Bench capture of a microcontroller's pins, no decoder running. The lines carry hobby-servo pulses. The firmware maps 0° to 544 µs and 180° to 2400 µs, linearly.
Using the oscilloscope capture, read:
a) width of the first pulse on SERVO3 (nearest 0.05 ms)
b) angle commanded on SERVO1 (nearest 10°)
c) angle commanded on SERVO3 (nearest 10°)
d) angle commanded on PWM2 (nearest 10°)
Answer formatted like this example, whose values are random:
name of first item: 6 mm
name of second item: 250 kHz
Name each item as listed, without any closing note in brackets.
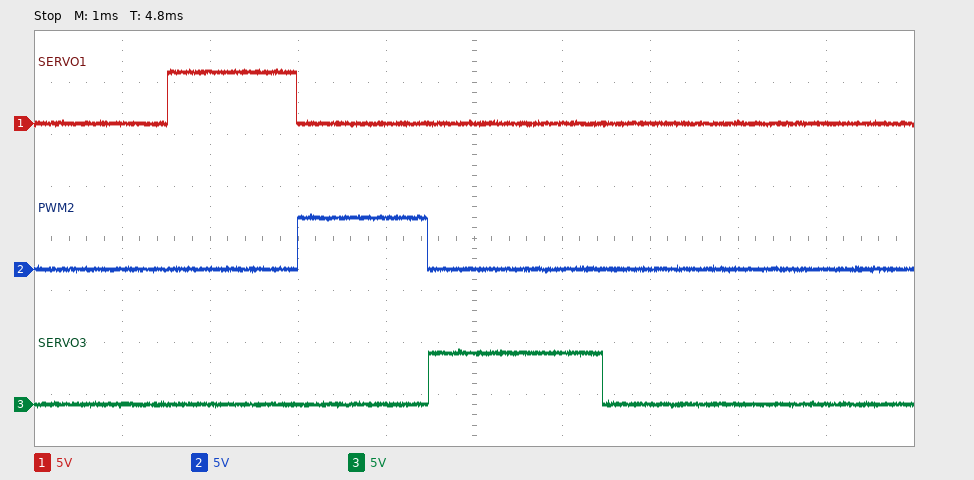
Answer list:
width of the first pulse on SERVO3: 2.00 ms
angle commanded on SERVO1: 90°
angle commanded on SERVO3: 140°
angle commanded on PWM2: 90°
